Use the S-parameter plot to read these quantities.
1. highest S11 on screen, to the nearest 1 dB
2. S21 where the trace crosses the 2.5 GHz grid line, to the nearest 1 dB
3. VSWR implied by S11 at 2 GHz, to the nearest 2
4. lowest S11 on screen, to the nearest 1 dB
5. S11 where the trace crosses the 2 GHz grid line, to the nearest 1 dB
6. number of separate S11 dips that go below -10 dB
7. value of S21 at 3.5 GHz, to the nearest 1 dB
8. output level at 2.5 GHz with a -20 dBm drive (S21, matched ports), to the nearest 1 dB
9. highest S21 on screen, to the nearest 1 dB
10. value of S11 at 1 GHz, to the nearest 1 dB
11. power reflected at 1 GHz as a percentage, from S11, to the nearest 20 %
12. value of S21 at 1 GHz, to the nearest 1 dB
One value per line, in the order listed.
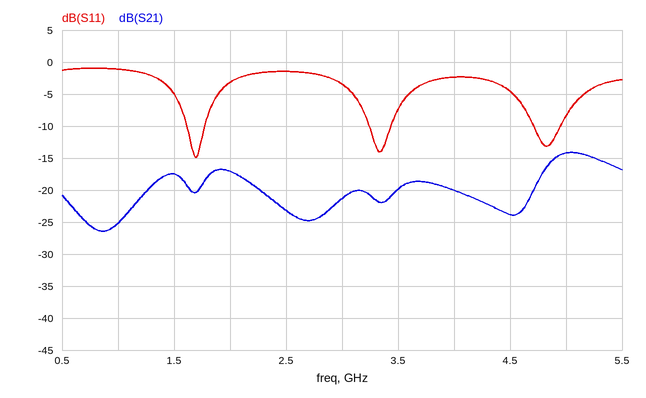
-1 dB
-23 dB
6
-15 dB
-3 dB
3
-20 dB
-43 dBm
-14 dB
-1 dB
80 %
-25 dB
